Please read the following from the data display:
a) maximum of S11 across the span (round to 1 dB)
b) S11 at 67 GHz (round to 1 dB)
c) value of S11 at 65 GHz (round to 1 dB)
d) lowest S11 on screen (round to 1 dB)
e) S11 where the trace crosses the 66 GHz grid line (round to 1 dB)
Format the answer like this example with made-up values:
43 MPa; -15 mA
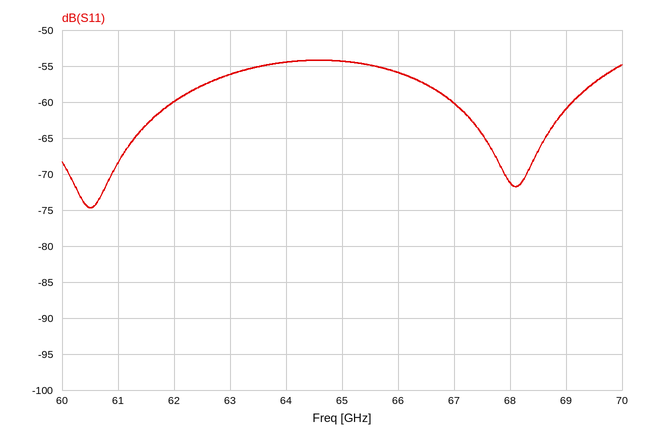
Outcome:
-54 dB; -60 dB; -54 dB; -75 dB; -56 dB
